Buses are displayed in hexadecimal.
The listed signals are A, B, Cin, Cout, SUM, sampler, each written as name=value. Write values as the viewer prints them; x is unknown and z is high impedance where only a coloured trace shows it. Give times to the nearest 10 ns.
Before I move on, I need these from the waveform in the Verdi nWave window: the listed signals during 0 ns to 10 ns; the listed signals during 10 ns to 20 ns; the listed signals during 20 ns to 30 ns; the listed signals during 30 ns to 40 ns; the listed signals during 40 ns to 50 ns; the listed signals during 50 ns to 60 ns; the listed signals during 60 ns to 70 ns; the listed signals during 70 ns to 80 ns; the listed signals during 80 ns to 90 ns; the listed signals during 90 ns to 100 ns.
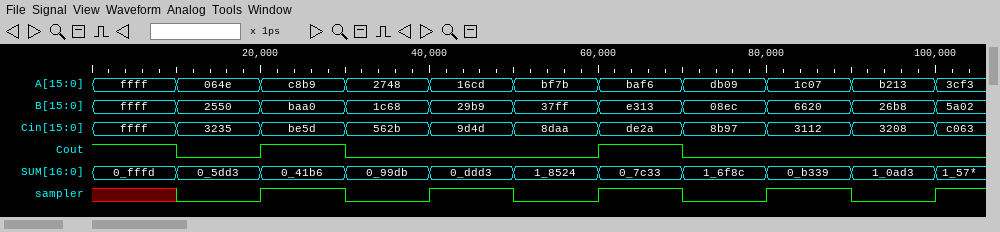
A=ffff, B=ffff, Cin=ffff, Cout=1, SUM=0_fffd, sampler=x
A=064e, B=2550, Cin=3235, Cout=0, SUM=0_5dd3, sampler=0
A=c8b9, B=baa0, Cin=be5d, Cout=1, SUM=0_41b6, sampler=1
A=2748, B=1c68, Cin=562b, Cout=0, SUM=0_99db, sampler=0
A=16cd, B=29b9, Cin=9d4d, Cout=0, SUM=0_ddd3, sampler=1
A=bf7b, B=37ff, Cin=8daa, Cout=0, SUM=1_8524, sampler=0
A=baf6, B=e313, Cin=de2a, Cout=1, SUM=0_7c33, sampler=1
A=db09, B=08ec, Cin=8b97, Cout=0, SUM=1_6f8c, sampler=0
A=1c07, B=6620, Cin=3112, Cout=0, SUM=0_b339, sampler=1
A=b213, B=26b8, Cin=3208, Cout=0, SUM=1_0ad3, sampler=0
